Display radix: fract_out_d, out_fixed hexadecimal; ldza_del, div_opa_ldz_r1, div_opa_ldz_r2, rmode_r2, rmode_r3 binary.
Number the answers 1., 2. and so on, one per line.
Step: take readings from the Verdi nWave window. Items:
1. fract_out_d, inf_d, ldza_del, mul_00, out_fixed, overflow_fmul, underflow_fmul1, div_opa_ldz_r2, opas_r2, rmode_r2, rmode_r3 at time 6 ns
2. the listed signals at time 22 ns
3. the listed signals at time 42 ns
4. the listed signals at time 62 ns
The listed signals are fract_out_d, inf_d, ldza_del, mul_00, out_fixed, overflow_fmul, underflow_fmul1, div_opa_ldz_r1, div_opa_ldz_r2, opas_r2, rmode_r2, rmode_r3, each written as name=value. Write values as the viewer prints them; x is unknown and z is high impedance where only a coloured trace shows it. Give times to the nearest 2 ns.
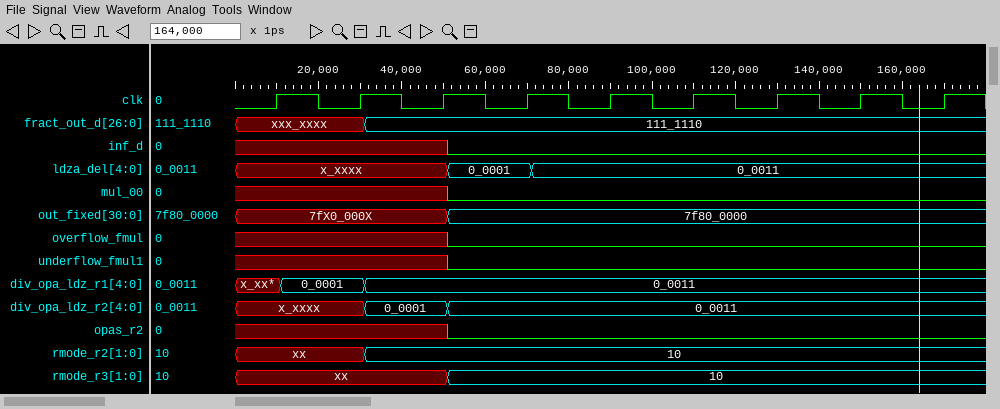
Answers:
1. fract_out_d=xxx_xxxx, inf_d=x, ldza_del=x_xxxx, mul_00=x, out_fixed=7fX0_000X, overflow_fmul=x, underflow_fmul1=x, div_opa_ldz_r2=x_xxxx, opas_r2=x, rmode_r2=xx, rmode_r3=xx
2. fract_out_d=xxx_xxxx, inf_d=x, ldza_del=x_xxxx, mul_00=x, out_fixed=7fX0_000X, overflow_fmul=x, underflow_fmul1=x, div_opa_ldz_r1=0_0001, div_opa_ldz_r2=x_xxxx, opas_r2=x, rmode_r2=xx, rmode_r3=xx
3. fract_out_d=111_1110, inf_d=x, ldza_del=x_xxxx, mul_00=x, out_fixed=7fX0_000X, overflow_fmul=x, underflow_fmul1=x, div_opa_ldz_r1=0_0011, div_opa_ldz_r2=0_0001, opas_r2=x, rmode_r2=10, rmode_r3=xx
4. fract_out_d=111_1110, inf_d=0, ldza_del=0_0001, mul_00=0, out_fixed=7f80_0000, overflow_fmul=0, underflow_fmul1=0, div_opa_ldz_r1=0_0011, div_opa_ldz_r2=0_0011, opas_r2=0, rmode_r2=10, rmode_r3=10
